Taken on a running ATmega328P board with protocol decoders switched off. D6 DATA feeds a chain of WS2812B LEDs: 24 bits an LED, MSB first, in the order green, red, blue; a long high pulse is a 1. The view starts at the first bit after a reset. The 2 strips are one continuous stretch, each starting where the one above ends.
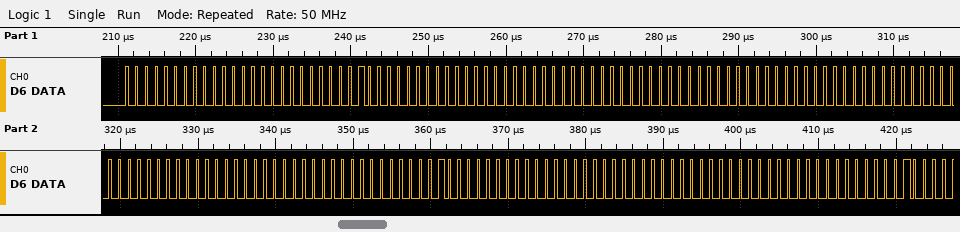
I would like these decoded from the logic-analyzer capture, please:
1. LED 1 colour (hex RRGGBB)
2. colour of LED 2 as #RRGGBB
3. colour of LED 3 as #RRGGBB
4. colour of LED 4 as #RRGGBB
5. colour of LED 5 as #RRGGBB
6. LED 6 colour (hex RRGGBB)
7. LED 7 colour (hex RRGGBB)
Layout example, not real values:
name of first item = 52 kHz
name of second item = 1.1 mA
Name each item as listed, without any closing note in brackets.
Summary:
LED 1 colour = #000000
colour of LED 2 as #RRGGBB = #008000
colour of LED 3 as #RRGGBB = #000000
colour of LED 4 as #RRGGBB = #000000
colour of LED 5 as #RRGGBB = #000000
LED 6 colour = #008000
LED 7 colour = #000000
